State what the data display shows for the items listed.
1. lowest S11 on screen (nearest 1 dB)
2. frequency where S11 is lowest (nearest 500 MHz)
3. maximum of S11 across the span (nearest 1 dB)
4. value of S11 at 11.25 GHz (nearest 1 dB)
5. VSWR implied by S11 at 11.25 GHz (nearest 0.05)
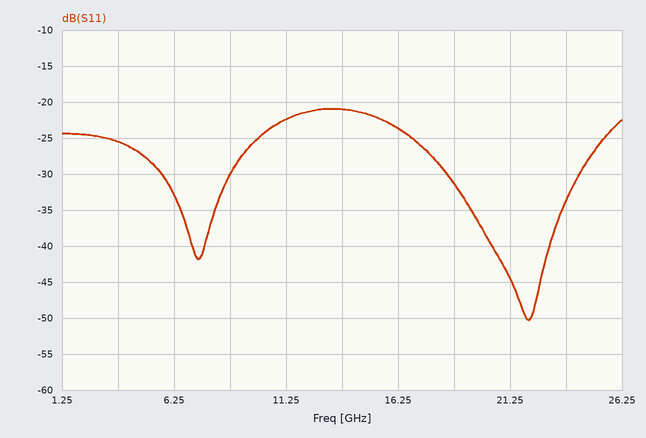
-50 dB
22.0 GHz
-21 dB
-22 dB
1.15
